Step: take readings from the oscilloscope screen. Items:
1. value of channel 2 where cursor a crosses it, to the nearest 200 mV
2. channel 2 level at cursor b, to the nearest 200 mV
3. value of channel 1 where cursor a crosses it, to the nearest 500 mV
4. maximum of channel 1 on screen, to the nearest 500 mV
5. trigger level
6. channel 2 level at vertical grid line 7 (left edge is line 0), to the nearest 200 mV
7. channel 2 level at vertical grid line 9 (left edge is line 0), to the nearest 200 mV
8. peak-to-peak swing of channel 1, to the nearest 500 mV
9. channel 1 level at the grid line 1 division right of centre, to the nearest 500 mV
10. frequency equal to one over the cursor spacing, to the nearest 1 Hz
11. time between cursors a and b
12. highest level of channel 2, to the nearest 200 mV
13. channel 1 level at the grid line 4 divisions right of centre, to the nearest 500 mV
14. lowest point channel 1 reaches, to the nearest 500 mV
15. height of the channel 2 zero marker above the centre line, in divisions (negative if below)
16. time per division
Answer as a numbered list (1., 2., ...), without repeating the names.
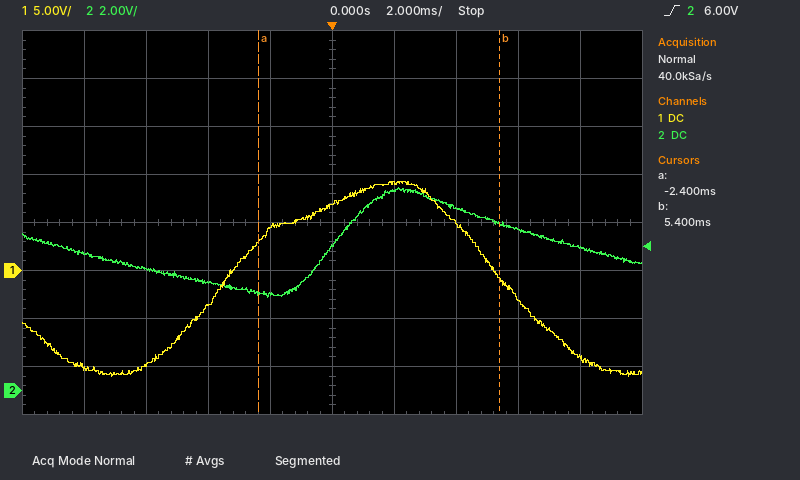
1. 4.0 V
2. 7.0 V
3. 3.0 V
4. 9.5 V
5. 6.00 V
6. 7.6 V
7. 6.0 V
8. 20.5 V
9. 9.0 V
10. 128 Hz
11. 7.8 ms
12. 8.4 V
13. -9.0 V
14. -11.0 V
15. -3.5 div
16. 2 ms
